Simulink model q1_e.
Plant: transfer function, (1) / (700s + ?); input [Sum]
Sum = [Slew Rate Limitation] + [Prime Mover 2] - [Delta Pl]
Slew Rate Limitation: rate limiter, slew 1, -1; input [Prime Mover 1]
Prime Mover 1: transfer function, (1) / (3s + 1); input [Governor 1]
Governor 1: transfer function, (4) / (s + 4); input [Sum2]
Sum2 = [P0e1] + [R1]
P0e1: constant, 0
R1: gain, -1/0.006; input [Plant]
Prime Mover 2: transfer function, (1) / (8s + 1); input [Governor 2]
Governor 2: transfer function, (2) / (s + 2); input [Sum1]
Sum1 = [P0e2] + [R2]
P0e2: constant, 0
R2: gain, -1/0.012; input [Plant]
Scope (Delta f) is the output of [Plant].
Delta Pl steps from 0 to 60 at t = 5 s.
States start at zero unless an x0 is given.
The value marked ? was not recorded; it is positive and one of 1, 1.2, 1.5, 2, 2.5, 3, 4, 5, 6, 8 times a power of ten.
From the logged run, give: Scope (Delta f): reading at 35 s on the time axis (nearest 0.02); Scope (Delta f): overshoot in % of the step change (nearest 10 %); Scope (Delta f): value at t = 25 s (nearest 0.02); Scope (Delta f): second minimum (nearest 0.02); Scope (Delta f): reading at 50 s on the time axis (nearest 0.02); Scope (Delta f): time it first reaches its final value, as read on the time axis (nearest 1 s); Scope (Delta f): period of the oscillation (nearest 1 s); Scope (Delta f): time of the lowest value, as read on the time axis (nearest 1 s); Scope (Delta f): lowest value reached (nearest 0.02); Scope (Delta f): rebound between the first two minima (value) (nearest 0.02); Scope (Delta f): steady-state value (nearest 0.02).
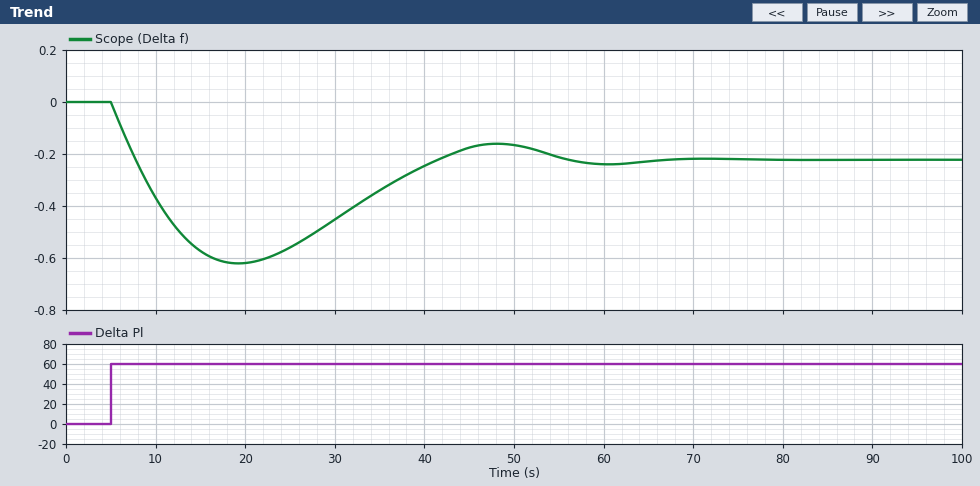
-0.34
180 %
-0.56
-0.24
-0.16
8 s
41 s
19 s
-0.62
-0.16
-0.22
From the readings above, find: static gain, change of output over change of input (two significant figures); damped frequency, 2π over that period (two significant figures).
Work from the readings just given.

-0.0037
0.15 rad/s
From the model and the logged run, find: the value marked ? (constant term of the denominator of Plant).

20
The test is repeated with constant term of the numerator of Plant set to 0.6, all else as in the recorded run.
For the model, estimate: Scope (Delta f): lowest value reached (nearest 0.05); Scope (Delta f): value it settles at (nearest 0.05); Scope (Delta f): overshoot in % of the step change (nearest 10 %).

-0.45
-0.20
110 %
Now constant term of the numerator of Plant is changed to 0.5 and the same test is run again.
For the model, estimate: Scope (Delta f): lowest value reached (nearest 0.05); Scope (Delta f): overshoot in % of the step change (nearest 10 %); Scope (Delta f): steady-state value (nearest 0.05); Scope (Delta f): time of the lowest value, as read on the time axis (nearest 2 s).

-0.40
90 %
-0.20
24 s
